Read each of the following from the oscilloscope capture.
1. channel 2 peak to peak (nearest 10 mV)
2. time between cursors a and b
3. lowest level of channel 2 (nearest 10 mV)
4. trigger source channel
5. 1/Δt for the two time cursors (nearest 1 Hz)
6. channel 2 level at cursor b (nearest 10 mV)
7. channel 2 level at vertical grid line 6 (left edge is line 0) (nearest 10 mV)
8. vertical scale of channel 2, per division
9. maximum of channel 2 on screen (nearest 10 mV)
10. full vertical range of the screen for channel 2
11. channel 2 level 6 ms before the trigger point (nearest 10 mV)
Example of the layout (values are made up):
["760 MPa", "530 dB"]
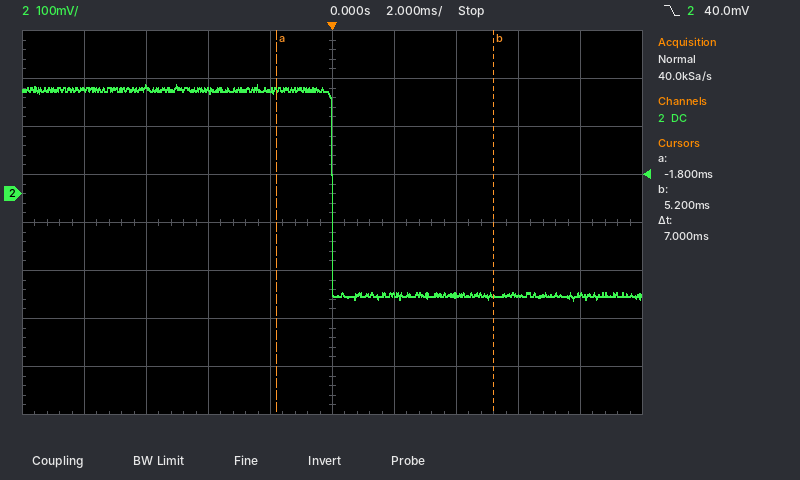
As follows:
["450 mV", "7 ms", "-220 mV", "channel 2", "143 Hz", "-210 mV", "-210 mV", "100 mV", "230 mV", "800 mV", "220 mV"]
